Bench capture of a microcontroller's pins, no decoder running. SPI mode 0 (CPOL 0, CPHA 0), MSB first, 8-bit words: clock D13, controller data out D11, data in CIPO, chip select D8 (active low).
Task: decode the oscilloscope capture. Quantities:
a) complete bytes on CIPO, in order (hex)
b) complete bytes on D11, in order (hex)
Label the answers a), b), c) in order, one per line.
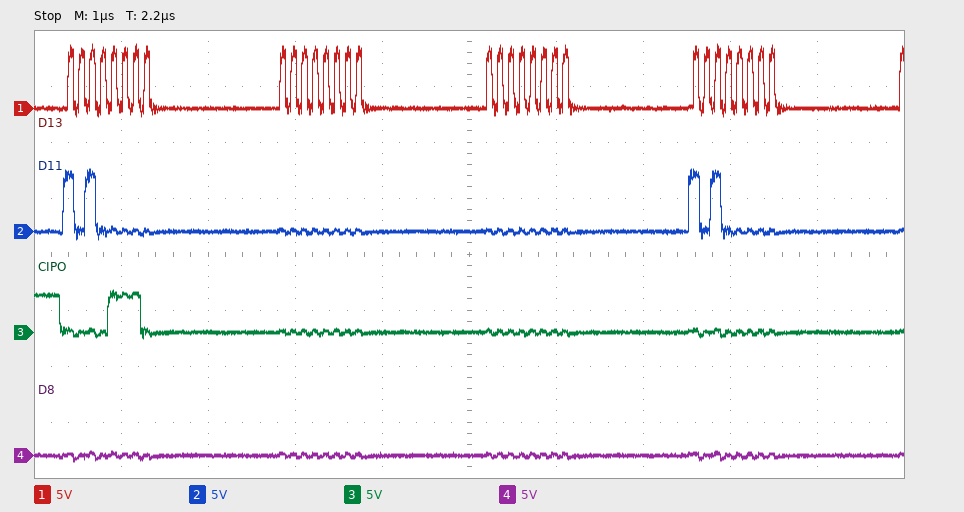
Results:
a) 0E 00 00 00
b) A0 00 00 A0
